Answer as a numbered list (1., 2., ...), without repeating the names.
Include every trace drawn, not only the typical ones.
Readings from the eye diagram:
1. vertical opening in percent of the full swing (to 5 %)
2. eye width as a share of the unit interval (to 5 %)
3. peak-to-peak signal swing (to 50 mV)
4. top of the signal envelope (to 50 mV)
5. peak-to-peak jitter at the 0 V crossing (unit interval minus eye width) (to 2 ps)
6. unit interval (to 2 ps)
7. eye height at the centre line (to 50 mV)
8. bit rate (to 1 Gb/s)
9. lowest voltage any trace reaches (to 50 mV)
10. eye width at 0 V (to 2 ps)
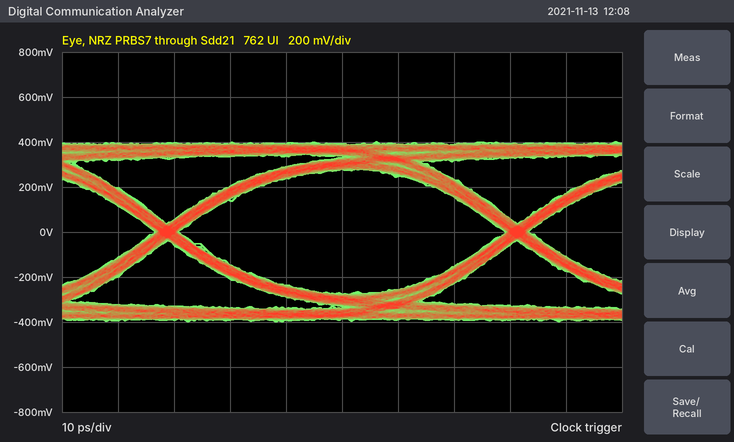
1. 70 %
2. 95 %
3. 800 mV
4. 400 mV
5. 4 ps
6. 62 ps
7. 550 mV
8. 16 Gb/s
9. -400 mV
10. 58 ps
